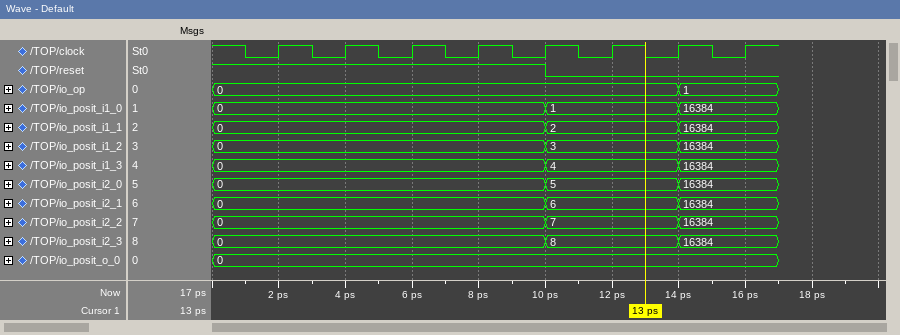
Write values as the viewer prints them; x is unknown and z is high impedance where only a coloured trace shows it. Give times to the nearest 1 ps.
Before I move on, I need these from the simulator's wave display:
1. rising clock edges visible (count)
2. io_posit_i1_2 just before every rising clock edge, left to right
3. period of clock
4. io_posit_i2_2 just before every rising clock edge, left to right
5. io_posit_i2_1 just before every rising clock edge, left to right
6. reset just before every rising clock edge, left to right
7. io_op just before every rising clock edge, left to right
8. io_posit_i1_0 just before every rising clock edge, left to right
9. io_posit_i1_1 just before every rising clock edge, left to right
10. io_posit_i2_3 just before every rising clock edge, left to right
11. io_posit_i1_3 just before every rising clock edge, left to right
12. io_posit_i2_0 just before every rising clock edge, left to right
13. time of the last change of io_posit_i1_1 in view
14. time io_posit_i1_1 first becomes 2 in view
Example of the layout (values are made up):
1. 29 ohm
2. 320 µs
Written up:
1. 8
2. 0, 0, 0, 0, 0, 3, 3, 16384
3. 2 ps
4. 0, 0, 0, 0, 0, 7, 7, 16384
5. 0, 0, 0, 0, 0, 6, 6, 16384
6. 1 1 1 1 1 0 0 0
7. 0, 0, 0, 0, 0, 0, 0, 1
8. 0, 0, 0, 0, 0, 1, 1, 16384
9. 0, 0, 0, 0, 0, 2, 2, 16384
10. 0, 0, 0, 0, 0, 8, 8, 16384
11. 0, 0, 0, 0, 0, 4, 4, 16384
12. 0, 0, 0, 0, 0, 5, 5, 16384
13. 14 ps
14. 10 ps
